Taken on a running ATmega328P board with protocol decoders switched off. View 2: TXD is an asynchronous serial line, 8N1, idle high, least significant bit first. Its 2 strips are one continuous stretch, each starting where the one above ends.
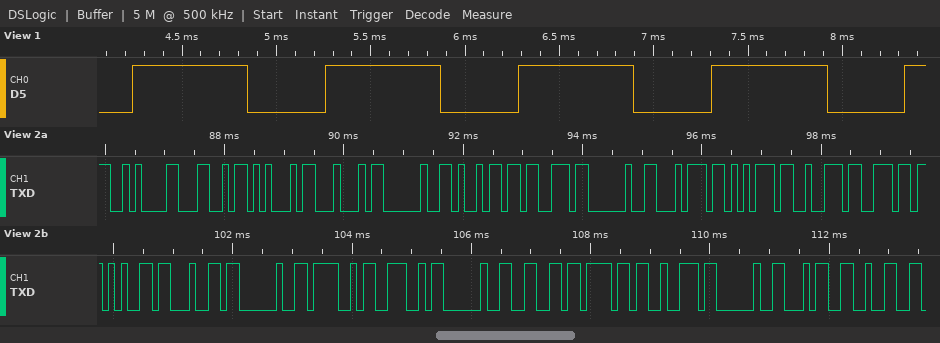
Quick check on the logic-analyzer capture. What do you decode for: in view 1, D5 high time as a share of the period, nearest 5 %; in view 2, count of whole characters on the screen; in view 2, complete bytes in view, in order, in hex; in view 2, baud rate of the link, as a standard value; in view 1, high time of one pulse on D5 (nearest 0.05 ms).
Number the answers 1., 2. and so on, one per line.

1. 60 %
2. 24
3. 0A 4C 45 44 20 69 73 20 74 75 72 6E 65 64 20 4F 4E 20 66 6F 72 20 34 32
4. 9600 baud
5. 0.60 ms
